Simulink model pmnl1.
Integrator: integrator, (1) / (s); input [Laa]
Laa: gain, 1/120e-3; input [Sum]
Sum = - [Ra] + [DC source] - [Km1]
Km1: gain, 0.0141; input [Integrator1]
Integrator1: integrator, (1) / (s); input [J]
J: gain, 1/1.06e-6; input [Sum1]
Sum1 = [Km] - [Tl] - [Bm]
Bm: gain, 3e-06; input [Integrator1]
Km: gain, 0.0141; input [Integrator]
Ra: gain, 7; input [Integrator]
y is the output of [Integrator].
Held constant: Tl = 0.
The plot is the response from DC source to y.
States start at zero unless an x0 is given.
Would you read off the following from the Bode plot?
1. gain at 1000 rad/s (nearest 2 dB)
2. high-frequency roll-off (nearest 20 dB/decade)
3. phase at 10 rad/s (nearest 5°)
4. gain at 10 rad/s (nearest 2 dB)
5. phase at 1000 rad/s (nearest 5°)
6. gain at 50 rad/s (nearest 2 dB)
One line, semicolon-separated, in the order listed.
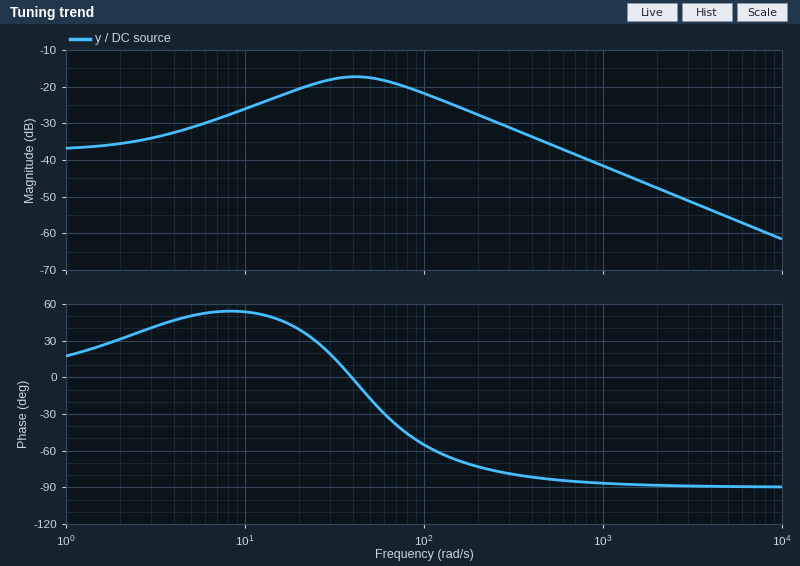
-42 dB; -20 dB/decade; 55°; -26 dB; -85°; -18 dB
